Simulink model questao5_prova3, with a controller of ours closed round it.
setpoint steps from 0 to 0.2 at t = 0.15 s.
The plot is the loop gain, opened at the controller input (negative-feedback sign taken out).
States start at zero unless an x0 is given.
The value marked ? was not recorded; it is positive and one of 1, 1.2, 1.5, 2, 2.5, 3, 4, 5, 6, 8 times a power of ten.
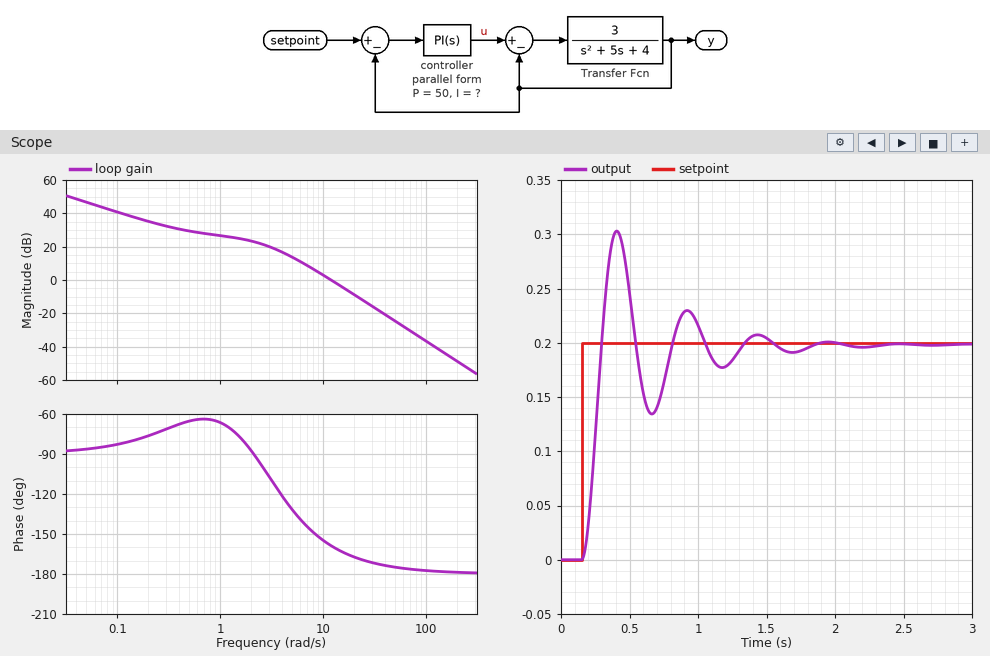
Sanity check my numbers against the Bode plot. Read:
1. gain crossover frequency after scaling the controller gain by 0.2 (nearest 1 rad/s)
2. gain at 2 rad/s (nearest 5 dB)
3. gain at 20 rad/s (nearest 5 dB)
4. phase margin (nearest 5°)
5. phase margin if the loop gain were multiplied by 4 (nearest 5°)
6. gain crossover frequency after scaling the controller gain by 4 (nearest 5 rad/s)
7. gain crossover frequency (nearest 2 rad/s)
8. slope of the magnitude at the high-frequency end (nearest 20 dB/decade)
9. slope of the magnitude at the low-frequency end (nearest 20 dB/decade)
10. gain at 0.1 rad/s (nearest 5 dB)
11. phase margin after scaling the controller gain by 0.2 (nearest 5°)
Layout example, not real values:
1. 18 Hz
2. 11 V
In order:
1. 5 rad/s
2. 25 dB
3. -10 dB
4. 20°
5. 10°
6. 25 rad/s
7. 12 rad/s
8. -40 dB/decade
9. -20 dB/decade
10. 40 dB
11. 50°
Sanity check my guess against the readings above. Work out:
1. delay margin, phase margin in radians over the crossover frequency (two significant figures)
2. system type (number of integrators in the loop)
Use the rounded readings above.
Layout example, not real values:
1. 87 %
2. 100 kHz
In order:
1. 0.029 s
2. 1
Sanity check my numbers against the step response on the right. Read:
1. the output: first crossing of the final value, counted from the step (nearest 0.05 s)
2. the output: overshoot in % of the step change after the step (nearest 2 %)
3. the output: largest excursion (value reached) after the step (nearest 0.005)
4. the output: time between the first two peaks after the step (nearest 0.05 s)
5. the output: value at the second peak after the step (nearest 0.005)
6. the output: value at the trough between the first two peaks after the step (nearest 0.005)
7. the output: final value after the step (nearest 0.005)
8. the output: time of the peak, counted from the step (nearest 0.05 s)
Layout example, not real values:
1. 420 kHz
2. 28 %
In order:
1. 0.15 s
2. 52 %
3. 0.305
4. 0.50 s
5. 0.230
6. 0.135
7. 0.200
8. 0.25 s
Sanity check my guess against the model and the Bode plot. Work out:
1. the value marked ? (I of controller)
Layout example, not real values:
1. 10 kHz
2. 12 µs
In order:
1. 25
